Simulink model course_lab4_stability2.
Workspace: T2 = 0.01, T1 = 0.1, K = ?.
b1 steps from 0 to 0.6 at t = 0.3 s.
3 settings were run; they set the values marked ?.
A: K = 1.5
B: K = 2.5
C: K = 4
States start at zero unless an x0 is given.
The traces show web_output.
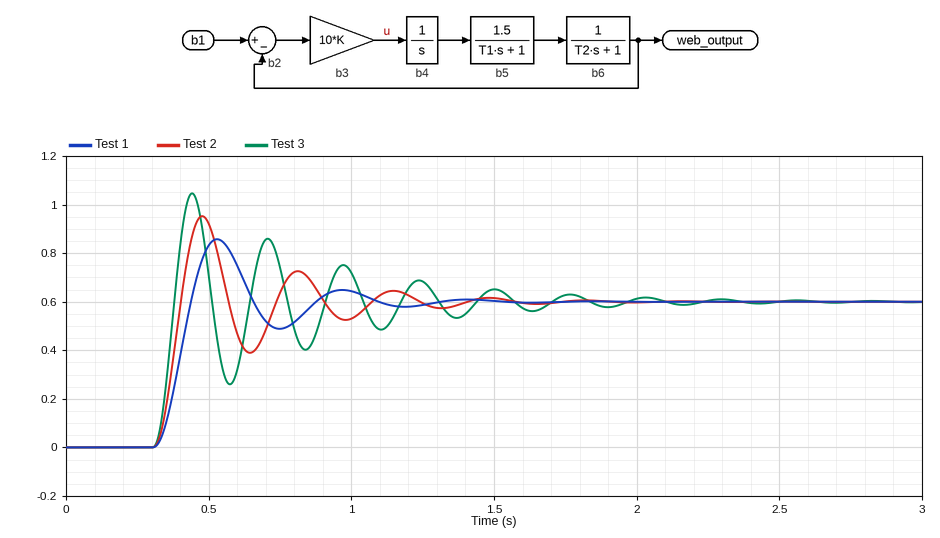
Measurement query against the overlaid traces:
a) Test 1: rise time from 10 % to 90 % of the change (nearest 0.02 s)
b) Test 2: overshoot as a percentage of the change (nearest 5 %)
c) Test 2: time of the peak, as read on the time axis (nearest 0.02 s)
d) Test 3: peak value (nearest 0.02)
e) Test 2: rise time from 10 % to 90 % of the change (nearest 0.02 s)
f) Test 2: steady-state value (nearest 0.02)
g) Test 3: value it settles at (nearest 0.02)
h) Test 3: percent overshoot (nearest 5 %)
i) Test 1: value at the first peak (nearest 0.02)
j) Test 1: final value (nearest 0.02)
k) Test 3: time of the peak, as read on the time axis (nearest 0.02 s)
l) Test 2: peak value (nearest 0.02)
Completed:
0.08 s
60 %
0.48 s
1.04
0.06 s
0.60
0.60
75 %
0.86
0.60
0.44 s
0.96
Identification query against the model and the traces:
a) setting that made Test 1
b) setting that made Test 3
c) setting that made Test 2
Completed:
A
C
B
